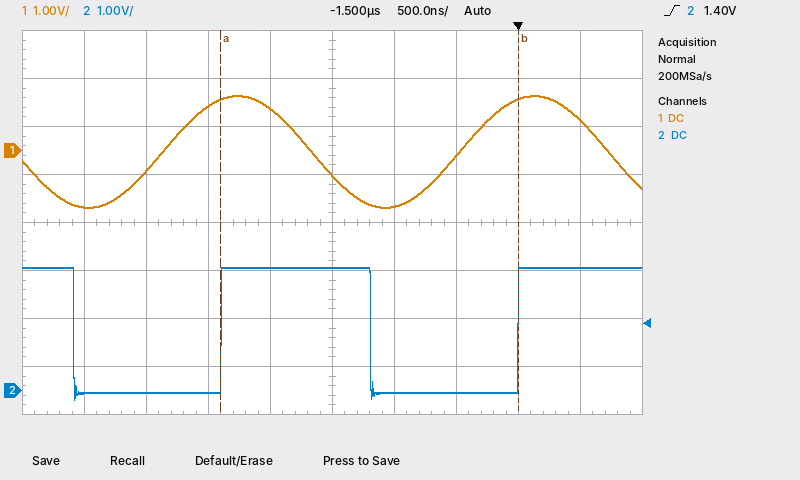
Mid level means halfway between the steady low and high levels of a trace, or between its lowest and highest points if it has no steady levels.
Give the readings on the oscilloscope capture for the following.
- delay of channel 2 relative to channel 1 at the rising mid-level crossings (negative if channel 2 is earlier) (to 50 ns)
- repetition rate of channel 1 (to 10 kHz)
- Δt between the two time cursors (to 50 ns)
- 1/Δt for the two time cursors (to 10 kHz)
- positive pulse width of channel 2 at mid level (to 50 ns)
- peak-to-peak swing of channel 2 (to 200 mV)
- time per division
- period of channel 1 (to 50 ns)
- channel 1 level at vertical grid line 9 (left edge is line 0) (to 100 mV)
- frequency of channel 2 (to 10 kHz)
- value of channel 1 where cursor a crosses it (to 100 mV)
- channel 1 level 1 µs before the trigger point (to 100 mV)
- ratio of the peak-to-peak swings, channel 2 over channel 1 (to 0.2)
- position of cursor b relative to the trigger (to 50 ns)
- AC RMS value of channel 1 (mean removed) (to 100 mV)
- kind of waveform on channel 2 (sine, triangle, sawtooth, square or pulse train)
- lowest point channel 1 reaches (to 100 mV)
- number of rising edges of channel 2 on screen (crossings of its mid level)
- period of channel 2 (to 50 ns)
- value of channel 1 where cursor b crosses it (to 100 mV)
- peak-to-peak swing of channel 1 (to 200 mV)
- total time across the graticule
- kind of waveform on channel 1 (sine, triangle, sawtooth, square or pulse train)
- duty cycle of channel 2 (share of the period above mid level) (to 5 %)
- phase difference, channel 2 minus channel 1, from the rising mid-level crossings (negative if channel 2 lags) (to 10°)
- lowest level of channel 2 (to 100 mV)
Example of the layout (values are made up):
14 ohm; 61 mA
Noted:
+450 ns; 420 kHz; 2.40 µs; 420 kHz; 1.20 µs; 2.8 V; 500 ns; 2.40 µs; 600 mV; 420 kHz; 1.1 V; -1.2 V; 1.2; 0 ns; 800 mV; square; -1.2 V; 2; 2.40 µs; 1.1 V; 2.4 V; 5 µs; sine; 50 %; -70°; -200 mV
